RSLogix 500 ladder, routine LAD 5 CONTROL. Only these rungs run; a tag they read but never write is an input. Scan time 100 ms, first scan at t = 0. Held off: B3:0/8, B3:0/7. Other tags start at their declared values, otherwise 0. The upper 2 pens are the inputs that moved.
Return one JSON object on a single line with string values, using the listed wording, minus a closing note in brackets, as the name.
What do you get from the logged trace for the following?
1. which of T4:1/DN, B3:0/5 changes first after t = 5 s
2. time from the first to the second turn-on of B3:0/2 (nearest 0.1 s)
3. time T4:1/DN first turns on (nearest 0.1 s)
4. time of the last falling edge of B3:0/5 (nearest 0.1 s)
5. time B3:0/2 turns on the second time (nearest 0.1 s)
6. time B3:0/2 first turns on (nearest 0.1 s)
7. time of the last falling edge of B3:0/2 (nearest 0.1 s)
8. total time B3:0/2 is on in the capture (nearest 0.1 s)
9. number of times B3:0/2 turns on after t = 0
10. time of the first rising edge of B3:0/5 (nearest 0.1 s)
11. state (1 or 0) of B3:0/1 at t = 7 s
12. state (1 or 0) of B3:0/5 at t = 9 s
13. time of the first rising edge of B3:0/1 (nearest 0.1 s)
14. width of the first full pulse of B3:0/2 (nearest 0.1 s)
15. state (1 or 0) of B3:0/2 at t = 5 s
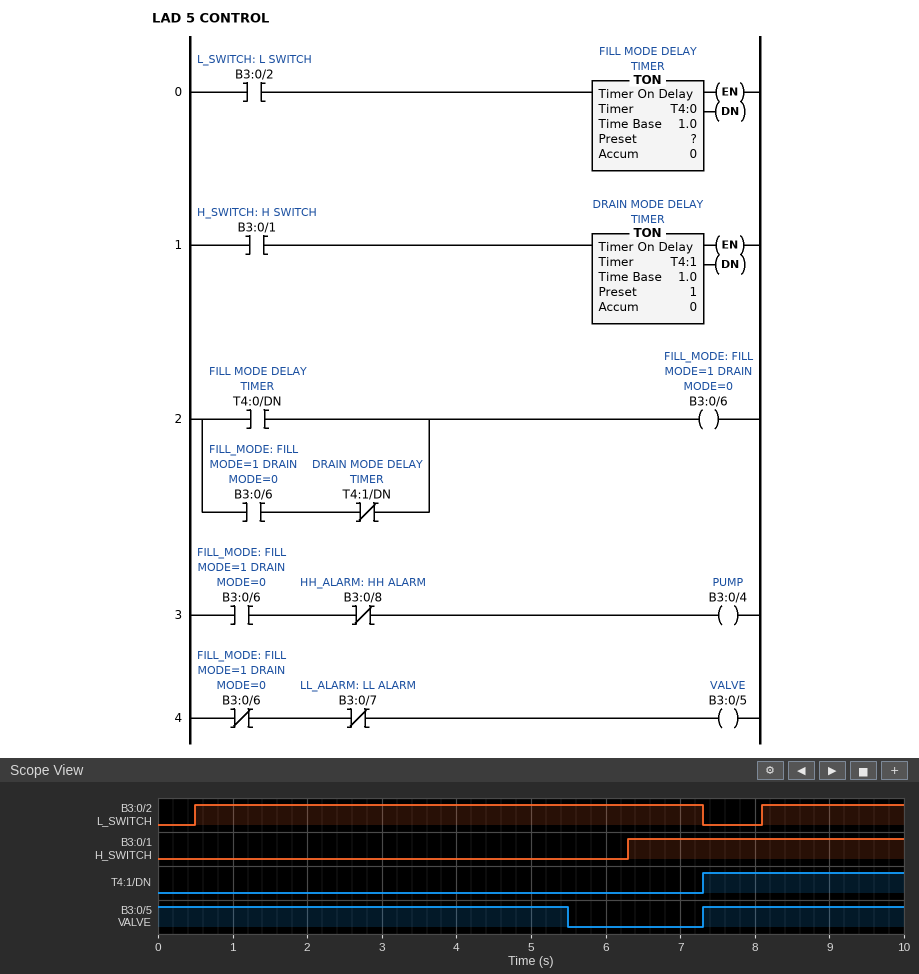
{"which of T4:1/DN, B3:0/5 changes first after t = 5 s": "B3:0/5", "time from the first to the second turn-on of B3:0/2": "7.6 s", "time T4:1/DN first turns on": "7.3 s", "time of the last falling edge of B3:0/5": "5.5 s", "time B3:0/2 turns on the second time": "8.1 s", "time B3:0/2 first turns on": "0.5 s", "time of the last falling edge of B3:0/2": "7.3 s", "total time B3:0/2 is on in the capture": "8.7 s", "number of times B3:0/2 turns on after t = 0": "2", "time of the first rising edge of B3:0/5": "7.3 s", "state (1 or 0) of B3:0/1 at t = 7 s": "1", "state (1 or 0) of B3:0/5 at t = 9 s": "1", "time of the first rising edge of B3:0/1": "6.3 s", "width of the first full pulse of B3:0/2": "6.8 s", "state (1 or 0) of B3:0/2 at t = 5 s": "1"}
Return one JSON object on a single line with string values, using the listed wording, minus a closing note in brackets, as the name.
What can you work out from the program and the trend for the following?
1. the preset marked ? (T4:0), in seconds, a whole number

{"the preset marked ? (T4:0), in seconds, a whole number": "5 s"}
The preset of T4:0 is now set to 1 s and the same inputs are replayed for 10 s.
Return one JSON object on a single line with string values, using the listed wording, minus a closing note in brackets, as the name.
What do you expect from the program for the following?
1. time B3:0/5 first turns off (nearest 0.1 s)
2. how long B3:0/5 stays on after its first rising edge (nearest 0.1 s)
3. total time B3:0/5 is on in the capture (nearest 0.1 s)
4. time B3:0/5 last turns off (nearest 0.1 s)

{"time B3:0/5 first turns off": "1.5 s", "how long B3:0/5 stays on after its first rising edge": "1.8 s", "total time B3:0/5 is on in the capture": "3.3 s", "time B3:0/5 last turns off": "9.1 s"}
